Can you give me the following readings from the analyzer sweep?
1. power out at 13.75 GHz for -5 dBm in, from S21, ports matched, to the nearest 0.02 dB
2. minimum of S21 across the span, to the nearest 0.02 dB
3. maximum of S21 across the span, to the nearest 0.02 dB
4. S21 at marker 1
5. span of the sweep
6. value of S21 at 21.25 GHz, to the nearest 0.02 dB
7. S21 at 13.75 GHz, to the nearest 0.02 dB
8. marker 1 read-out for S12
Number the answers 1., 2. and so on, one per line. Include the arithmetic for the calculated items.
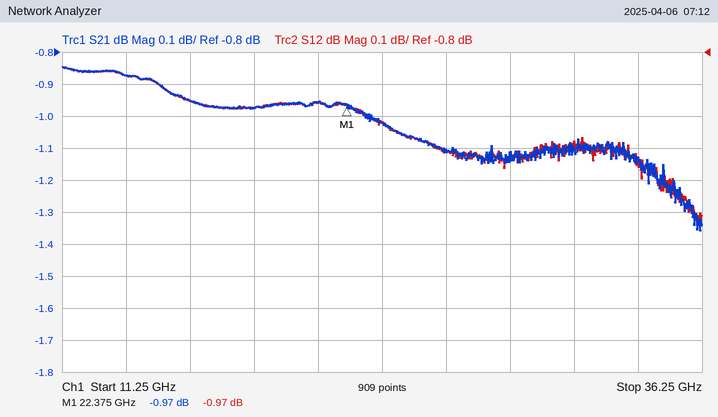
1. -5 dBm + (-0.88 dB) = -5.88 dBm
2. -1.36 dB
3. -0.84 dB
4. -0.97 dB
5. 25 GHz
6. -0.96 dB
7. -0.88 dB
8. -0.97 dB
